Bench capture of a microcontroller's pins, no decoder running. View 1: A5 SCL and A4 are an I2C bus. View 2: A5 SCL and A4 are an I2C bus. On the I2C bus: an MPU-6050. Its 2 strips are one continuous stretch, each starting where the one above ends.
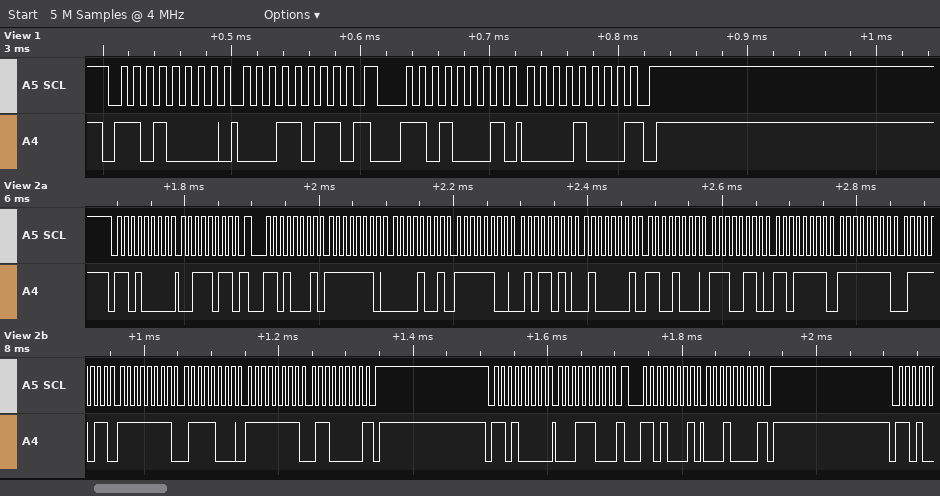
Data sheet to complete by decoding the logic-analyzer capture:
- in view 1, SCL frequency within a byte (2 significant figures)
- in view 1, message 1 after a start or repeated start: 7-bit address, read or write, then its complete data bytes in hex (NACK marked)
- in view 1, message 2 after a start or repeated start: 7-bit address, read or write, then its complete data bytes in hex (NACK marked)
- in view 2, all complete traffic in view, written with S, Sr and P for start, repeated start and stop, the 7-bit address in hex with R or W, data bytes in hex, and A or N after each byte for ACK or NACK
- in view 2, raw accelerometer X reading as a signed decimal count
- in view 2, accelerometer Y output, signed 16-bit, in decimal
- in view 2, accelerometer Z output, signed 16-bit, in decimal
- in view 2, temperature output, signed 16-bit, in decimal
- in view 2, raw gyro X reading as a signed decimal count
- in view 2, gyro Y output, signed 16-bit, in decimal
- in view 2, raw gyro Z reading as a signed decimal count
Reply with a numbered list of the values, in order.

1. 100 kHz
2. 0x68 write: 1B
3. 0x68 read: 08 NACK
4. S 68W A 3B A Sr 68R A FE A 09 A FC A 5A A 41 A C8 A E6 A DF A FF A 7B A FF A 78 A FF A 60 N P S 68W A 1C A Sr 68R A 10 N P
5. -503
6. -934
7. 16840
8. -6433
9. -133
10. -136
11. -160
